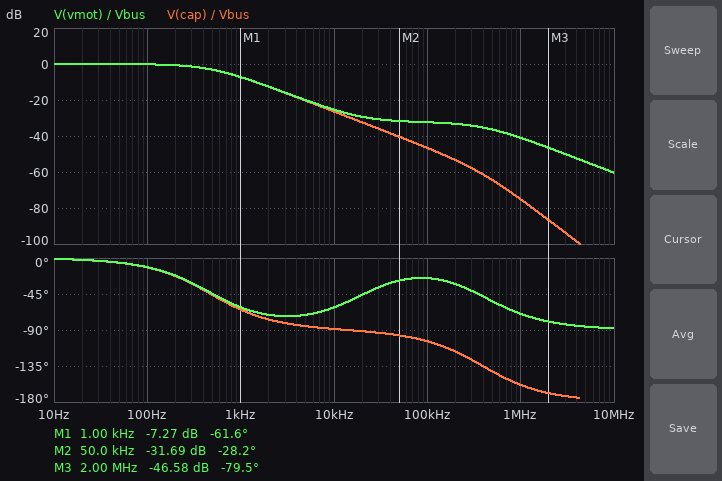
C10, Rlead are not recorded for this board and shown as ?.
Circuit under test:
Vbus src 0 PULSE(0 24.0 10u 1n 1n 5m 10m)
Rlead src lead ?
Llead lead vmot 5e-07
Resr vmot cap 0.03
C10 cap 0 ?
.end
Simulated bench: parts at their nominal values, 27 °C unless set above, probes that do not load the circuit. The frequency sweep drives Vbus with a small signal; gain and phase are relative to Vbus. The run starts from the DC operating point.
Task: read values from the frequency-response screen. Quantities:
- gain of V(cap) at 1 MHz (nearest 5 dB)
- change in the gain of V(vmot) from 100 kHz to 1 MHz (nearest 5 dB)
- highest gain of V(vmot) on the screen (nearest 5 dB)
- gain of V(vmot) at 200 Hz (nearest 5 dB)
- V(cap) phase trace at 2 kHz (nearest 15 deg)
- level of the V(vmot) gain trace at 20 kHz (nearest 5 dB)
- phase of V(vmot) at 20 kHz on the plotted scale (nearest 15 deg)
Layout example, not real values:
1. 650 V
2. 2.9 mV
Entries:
1. -75 dB
2. -10 dB
3. 0 dB
4. 0 dB
5. -75 deg
6. -30 dB
7. -45 deg
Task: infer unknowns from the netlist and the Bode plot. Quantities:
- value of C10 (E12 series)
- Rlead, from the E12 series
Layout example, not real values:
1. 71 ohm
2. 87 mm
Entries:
1. 270 µF
2. 1.2 Ω
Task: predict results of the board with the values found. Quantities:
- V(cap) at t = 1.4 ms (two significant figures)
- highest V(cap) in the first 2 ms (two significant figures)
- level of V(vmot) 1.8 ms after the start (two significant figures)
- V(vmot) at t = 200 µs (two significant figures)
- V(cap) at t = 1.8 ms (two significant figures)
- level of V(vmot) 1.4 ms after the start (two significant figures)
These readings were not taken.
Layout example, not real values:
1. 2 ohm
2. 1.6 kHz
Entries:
1. 24 V
2. 24 V
3. 24 V
4. 11 V
5. 24 V
6. 24 V
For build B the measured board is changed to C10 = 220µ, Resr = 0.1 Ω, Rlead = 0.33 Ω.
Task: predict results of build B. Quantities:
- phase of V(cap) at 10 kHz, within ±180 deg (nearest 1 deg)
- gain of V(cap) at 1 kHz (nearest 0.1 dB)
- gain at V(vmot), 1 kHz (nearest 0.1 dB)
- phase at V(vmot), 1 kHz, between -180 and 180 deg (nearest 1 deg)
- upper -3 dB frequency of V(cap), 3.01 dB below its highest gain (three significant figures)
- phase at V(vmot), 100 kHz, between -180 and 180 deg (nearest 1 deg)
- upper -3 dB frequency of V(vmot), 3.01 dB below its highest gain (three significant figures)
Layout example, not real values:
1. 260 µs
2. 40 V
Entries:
1. -85 deg
2. -1.3 dB
3. -1.2 dB
4. -23 deg
5. 1.70 kHz
6. -40 deg
7. 1.81 kHz
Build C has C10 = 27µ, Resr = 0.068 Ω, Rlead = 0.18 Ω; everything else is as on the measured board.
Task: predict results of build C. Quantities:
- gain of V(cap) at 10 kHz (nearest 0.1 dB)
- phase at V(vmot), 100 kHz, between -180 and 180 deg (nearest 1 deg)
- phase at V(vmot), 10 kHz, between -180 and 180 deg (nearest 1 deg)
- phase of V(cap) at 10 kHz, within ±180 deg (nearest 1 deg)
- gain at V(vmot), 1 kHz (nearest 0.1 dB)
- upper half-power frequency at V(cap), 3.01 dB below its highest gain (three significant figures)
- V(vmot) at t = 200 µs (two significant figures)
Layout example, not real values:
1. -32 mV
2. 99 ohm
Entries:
1. -0.3 dB
2. -87 deg
3. -17 deg
4. -24 deg
5. 0 dB
6. 31.8 kHz
7. 24 V
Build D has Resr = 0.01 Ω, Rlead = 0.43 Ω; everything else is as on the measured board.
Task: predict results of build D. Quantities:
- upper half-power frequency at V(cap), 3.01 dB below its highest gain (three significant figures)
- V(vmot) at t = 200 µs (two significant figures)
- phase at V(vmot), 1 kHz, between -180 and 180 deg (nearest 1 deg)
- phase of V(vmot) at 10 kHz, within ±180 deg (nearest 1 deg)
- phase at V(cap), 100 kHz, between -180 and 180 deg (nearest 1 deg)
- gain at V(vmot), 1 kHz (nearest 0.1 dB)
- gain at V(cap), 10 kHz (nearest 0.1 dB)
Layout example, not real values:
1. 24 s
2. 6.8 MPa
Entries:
1. 1.35 kHz
2. 19 V
3. -36 deg
4. -77 deg
5. -125 deg
6. -1.9 dB
7. -17.5 dB
